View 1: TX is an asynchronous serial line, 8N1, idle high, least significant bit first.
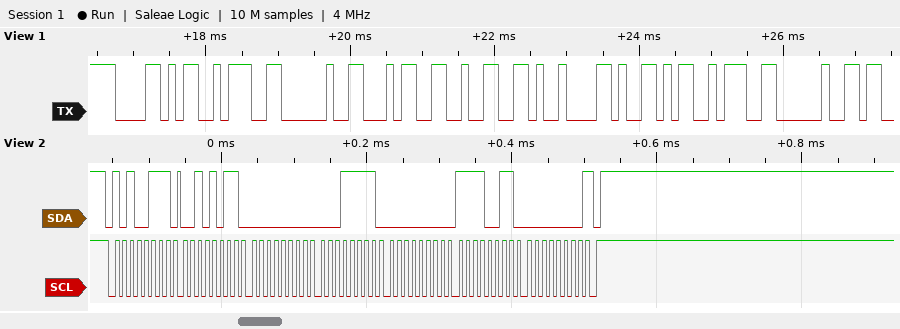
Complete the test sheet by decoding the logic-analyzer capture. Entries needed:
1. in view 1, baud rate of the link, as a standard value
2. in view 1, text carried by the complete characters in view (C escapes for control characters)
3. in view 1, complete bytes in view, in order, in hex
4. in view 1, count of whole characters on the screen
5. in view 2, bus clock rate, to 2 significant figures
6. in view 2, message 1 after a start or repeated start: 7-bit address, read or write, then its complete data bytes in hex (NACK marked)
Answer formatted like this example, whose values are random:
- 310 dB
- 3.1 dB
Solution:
- 9600 baud
- "X: 42\tY: "
- 58 3A 20 34 32 09 59 3A 20
- 9
- 100 kHz
- 0x53 read: 2B 00 1F 00 F3 00 NACK
